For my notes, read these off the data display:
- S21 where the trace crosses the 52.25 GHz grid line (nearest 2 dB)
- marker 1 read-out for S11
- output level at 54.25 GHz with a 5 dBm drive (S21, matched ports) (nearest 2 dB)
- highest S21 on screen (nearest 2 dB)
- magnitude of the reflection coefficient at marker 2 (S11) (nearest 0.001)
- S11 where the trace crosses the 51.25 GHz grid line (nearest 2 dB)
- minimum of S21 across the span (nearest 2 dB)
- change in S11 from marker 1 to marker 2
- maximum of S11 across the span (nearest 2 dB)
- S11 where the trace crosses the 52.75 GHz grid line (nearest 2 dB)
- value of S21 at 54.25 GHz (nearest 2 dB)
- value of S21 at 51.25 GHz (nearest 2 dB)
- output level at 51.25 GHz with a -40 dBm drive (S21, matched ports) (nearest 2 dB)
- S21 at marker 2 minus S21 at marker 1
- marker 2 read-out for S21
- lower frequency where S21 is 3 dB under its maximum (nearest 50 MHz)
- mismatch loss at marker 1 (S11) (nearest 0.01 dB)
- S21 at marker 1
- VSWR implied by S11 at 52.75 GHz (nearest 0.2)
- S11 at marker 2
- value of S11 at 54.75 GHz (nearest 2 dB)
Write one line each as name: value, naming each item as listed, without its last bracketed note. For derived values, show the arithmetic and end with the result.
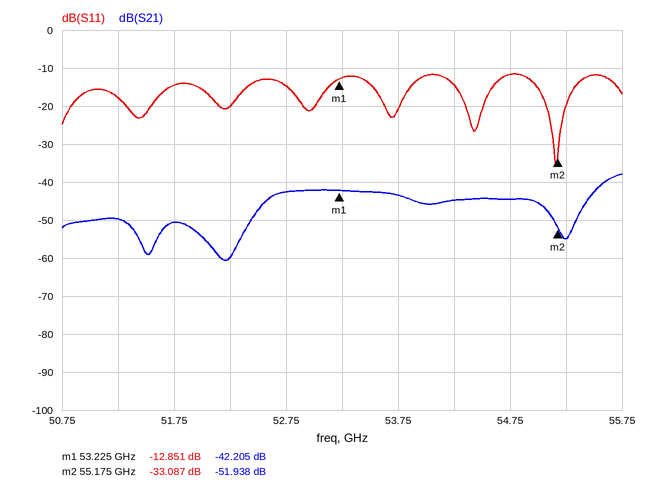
S21 where the trace crosses the 52.25 GHz grid line: -60 dB
marker 1 read-out for S11: -12.851 dB
output level at 54.25 GHz with a 5 dBm drive (S21, matched ports): 5 dBm + (-44 dB) = -40 dBm
highest S21 on screen: -38 dB
magnitude of the reflection coefficient at marker 2 (S11): 10^(-33.087/20) ≈ 0.022
S11 where the trace crosses the 51.25 GHz grid line: -18 dB
minimum of S21 across the span: -60 dB
change in S11 from marker 1 to marker 2: -33.087 − (-12.851) = -20.236 dB
maximum of S11 across the span: -12 dB
S11 where the trace crosses the 52.75 GHz grid line: -14 dB
value of S21 at 54.25 GHz: -44 dB
value of S21 at 51.25 GHz: -50 dB
output level at 51.25 GHz with a -40 dBm drive (S21, matched ports): -40 dBm + (-50 dB) = -90 dBm
S21 at marker 2 minus S21 at marker 1: -51.938 − (-42.205) = -9.733 dB
marker 2 read-out for S21: -51.938 dB
lower frequency where S21 is 3 dB under its maximum: 55.55 GHz
mismatch loss at marker 1 (S11): −10 log10(1 − 10^(-12.851/10)) ≈ 0.23 dB
S21 at marker 1: -42.205 dB
VSWR implied by S11 at 52.75 GHz: |Γ| = 10^(-14/20) = 0.1995; VSWR = (1 + 0.1995)/(1 − 0.1995) ≈ 1.50, so 1.4 to the nearest 0.2
S11 at marker 2: -33.087 dB
value of S11 at 54.75 GHz: -12 dB
